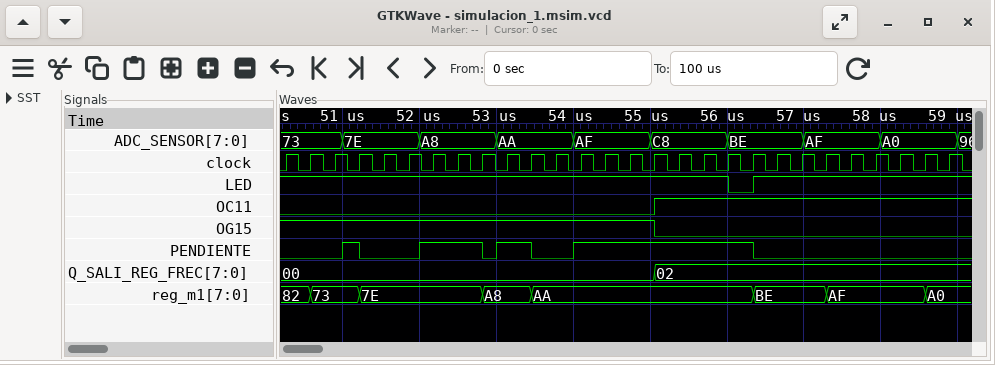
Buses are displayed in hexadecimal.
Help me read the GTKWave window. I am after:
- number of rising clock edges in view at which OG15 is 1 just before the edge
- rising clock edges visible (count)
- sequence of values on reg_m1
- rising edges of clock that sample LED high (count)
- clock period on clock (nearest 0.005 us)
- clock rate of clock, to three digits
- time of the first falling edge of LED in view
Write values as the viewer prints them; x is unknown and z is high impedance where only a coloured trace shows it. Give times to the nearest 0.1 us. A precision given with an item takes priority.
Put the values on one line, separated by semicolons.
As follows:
16; 28; 82, 73, 7E, A8, AA, BE, AF, A0; 27; 0.32 us; 3.12 MHz; 56 us
